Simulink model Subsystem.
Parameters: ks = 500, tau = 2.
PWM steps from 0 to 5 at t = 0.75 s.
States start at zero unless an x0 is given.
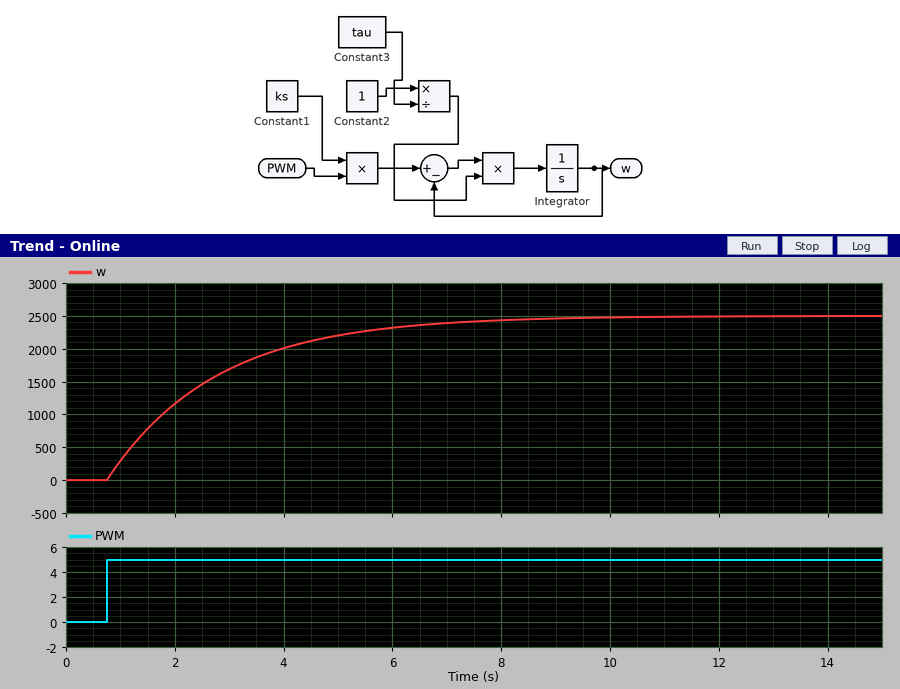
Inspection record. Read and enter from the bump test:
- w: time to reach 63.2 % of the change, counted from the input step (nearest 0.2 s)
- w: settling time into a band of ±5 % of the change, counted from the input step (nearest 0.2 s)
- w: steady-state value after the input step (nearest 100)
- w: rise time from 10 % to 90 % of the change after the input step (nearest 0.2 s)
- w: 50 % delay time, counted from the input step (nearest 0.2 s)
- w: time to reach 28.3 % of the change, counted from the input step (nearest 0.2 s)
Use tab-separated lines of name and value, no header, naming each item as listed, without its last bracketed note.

w: time to reach 63.2 % of the change, counted from the input step	2.0 s
w: settling time into a band of ±5 % of the change, counted from the input step	6.0 s
w: steady-state value after the input step	2500
w: rise time from 10 % to 90 % of the change after the input step	4.4 s
w: 50 % delay time, counted from the input step	1.4 s
w: time to reach 28.3 % of the change, counted from the input step	0.6 s
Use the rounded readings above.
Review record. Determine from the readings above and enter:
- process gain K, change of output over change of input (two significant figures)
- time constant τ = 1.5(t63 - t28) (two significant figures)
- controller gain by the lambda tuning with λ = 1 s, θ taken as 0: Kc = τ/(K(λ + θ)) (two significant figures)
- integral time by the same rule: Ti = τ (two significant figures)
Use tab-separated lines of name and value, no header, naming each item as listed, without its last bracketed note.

process gain K, change of output over change of input	500
time constant τ = 1.5(t63 - t28)	2.1 s
controller gain by the lambda tuning with λ = 1 s, θ taken as 0: Kc = τ/(K(λ + θ))	0.0042
integral time by the same rule: Ti = τ	2.1 s
